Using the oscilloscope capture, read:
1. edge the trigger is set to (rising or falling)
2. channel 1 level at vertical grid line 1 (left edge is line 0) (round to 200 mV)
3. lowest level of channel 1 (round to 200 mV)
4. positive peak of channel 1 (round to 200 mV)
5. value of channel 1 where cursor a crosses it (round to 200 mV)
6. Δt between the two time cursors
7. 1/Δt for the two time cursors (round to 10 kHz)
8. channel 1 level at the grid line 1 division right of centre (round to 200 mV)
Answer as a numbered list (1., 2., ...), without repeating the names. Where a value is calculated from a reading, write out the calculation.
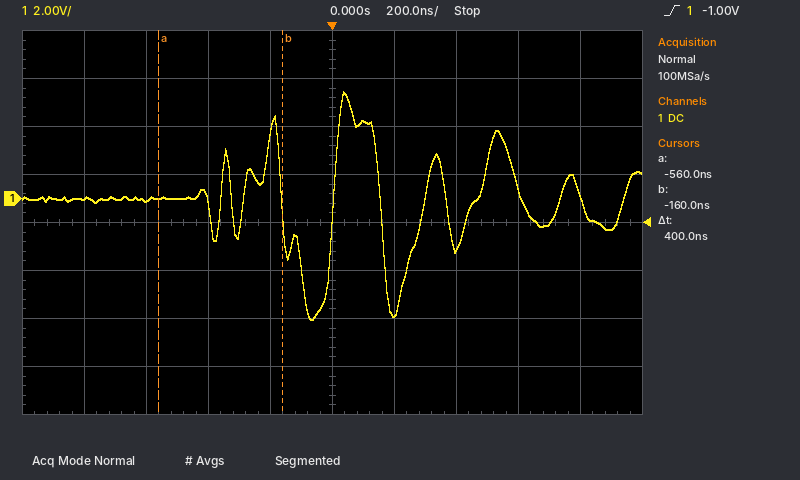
1. rising
2. 0.0 V
3. -5.0 V
4. 4.4 V
5. 0.0 V
6. 400 ns
7. 1 / 400 ns ≈ 2.50 MHz
8. -4.8 V
